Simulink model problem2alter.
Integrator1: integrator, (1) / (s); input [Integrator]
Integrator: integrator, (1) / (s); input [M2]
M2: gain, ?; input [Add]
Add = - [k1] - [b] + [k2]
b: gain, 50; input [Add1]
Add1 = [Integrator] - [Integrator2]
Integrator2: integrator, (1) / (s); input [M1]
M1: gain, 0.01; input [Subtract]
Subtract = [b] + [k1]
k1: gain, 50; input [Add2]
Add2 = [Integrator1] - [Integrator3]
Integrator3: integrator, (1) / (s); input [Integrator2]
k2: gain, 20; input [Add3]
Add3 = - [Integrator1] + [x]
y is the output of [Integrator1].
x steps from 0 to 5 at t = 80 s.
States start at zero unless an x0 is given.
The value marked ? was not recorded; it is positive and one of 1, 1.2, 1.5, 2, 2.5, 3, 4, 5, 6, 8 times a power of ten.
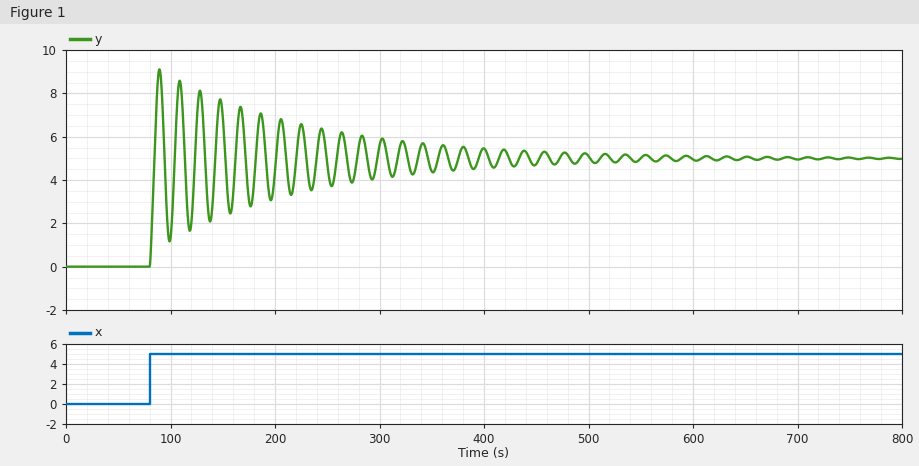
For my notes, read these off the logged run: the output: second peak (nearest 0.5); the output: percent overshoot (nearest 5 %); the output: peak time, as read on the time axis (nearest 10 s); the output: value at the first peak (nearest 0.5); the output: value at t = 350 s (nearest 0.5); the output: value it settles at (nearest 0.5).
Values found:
8.5
80 %
90 s
9.0
4.5
5.0
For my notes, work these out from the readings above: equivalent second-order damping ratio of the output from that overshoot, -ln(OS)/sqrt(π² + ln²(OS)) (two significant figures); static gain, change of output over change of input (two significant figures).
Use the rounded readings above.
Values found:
0.071
1.0
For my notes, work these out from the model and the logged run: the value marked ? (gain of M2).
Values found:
0.015
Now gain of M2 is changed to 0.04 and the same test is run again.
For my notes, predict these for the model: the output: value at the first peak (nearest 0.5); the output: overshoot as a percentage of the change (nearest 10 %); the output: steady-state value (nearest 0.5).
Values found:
8.5
70 %
5.0
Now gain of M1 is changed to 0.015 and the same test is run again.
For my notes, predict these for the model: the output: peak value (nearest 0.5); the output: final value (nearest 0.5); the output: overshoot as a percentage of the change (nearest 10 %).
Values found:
9.5
5.0
90 %
